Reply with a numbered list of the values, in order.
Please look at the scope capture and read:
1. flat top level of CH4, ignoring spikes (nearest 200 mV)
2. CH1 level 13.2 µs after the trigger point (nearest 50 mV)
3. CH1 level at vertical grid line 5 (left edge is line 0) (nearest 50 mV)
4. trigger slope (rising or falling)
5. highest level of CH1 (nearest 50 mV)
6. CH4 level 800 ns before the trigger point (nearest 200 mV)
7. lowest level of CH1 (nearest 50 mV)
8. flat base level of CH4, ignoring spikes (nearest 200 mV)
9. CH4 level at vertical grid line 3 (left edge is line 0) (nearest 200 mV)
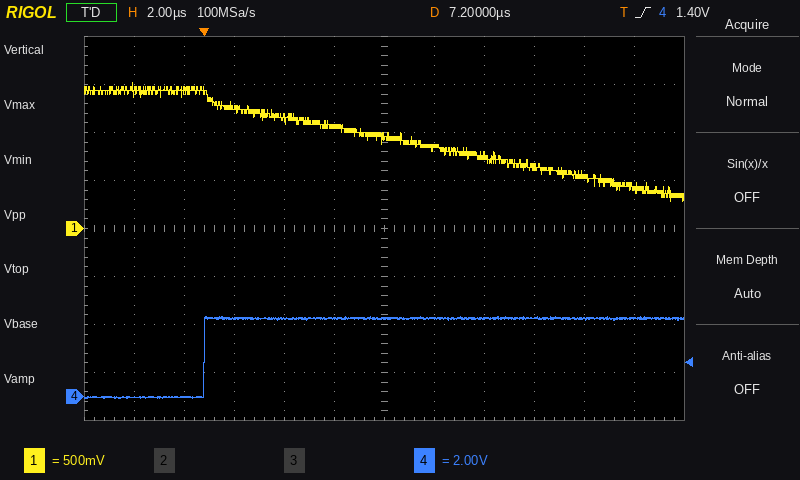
1. 3.2 V
2. 650 mV
3. 1.05 V
4. rising
5. 1.50 V
6. 0.0 V
7. 300 mV
8. 0.0 V
9. 3.2 V
